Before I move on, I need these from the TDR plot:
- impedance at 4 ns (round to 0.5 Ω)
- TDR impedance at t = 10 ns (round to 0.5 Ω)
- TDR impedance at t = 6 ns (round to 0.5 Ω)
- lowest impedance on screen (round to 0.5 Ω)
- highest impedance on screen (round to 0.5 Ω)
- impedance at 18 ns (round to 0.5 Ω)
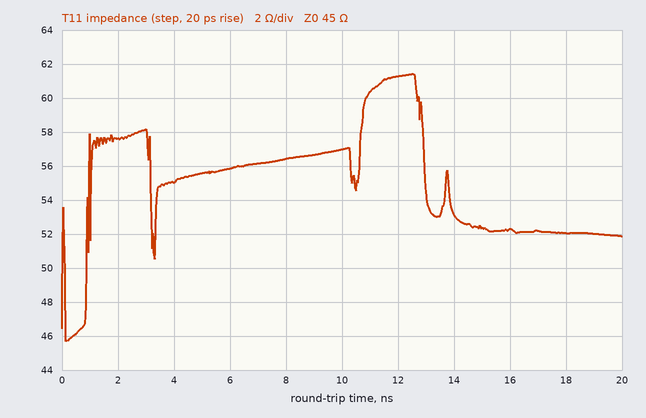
55.0 Ω
57.0 Ω
56.0 Ω
45.5 Ω
61.5 Ω
52.0 Ω
